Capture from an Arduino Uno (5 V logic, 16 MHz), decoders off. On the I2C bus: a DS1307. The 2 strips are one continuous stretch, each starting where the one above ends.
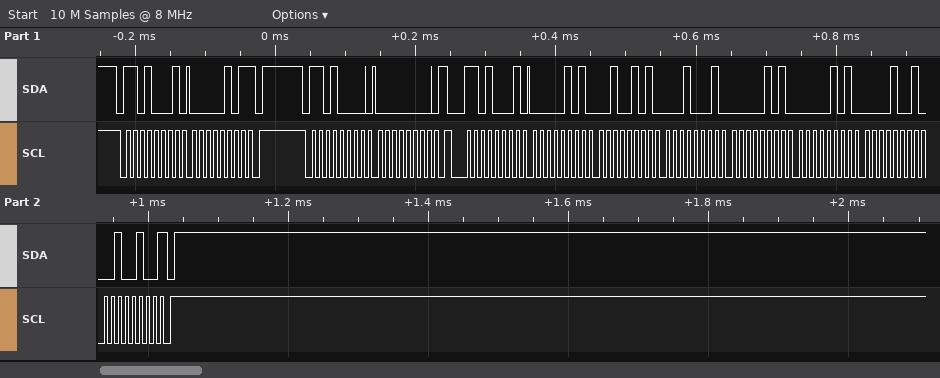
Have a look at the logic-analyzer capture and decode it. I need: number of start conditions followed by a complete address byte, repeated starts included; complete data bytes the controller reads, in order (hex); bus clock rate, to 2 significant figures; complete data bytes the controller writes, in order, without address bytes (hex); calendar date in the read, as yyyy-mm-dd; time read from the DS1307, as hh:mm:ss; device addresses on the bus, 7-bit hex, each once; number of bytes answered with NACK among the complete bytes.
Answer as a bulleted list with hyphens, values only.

- 3
- 05 05 25 11 05 05 09 24
- 100 kHz
- 00
- 2024-09-05
- 11:25:05
- 0x68
- 2
